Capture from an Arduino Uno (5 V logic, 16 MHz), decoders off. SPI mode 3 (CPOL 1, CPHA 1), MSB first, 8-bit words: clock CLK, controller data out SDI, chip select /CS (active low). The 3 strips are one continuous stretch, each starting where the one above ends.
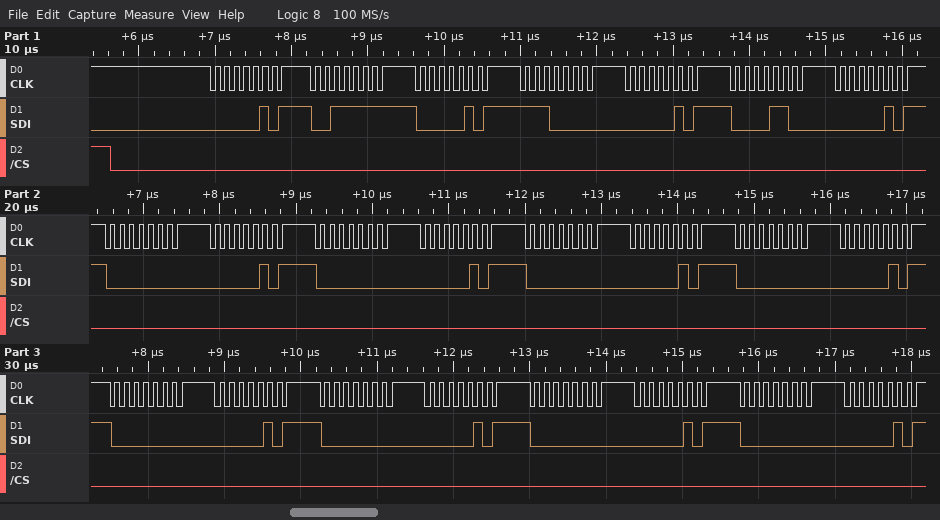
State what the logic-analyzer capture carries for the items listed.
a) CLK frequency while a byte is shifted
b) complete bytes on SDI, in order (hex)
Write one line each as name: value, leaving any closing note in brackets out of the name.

CLK frequency while a byte is shifted: 8 MHz
complete bytes on SDI, in order: 05 3F 05 E0 05 0C 05 00 05 00 05 00 05 00 05 00 05 00 05 00 05 00 05
